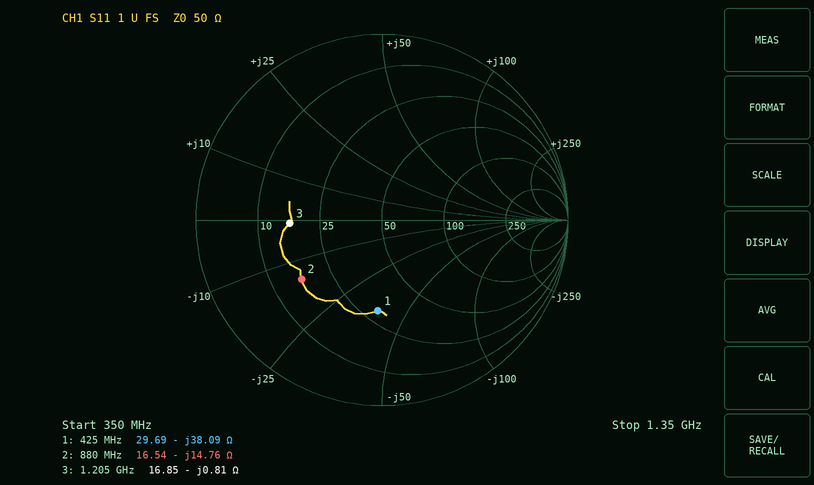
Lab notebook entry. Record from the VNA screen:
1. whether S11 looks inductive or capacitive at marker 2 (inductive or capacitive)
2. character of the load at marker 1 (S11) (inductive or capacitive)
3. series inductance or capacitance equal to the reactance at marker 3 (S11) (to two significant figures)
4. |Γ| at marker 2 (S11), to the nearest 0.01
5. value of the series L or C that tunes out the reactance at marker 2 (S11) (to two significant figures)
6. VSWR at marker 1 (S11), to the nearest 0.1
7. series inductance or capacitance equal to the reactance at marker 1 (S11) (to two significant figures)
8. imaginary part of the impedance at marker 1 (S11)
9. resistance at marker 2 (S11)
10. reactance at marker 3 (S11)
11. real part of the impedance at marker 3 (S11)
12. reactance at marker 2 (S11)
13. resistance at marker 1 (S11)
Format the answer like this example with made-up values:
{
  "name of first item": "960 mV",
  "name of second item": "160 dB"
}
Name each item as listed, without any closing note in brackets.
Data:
{
  "whether S11 looks inductive or capacitive at marker 2": "capacitive",
  "character of the load at marker 1 (S11)": "capacitive",
  "series inductance or capacitance equal to the reactance at marker 3 (S11)": "160 pF",
  "|Γ| at marker 2 (S11), to the nearest 0.01": "0.54",
  "value of the series L or C that tunes out the reactance at marker 2 (S11)": "2.7 nH",
  "VSWR at marker 1 (S11), to the nearest 0.1": "2.9",
  "series inductance or capacitance equal to the reactance at marker 1 (S11)": "9.8 pF",
  "imaginary part of the impedance at marker 1": "-38.09 Ω",
  "resistance at marker 2": "16.54 Ω",
  "reactance at marker 3": "-0.81 Ω",
  "real part of the impedance at marker 3": "16.85 Ω",
  "reactance at marker 2": "-14.76 Ω",
  "resistance at marker 1": "29.69 Ω"
}
